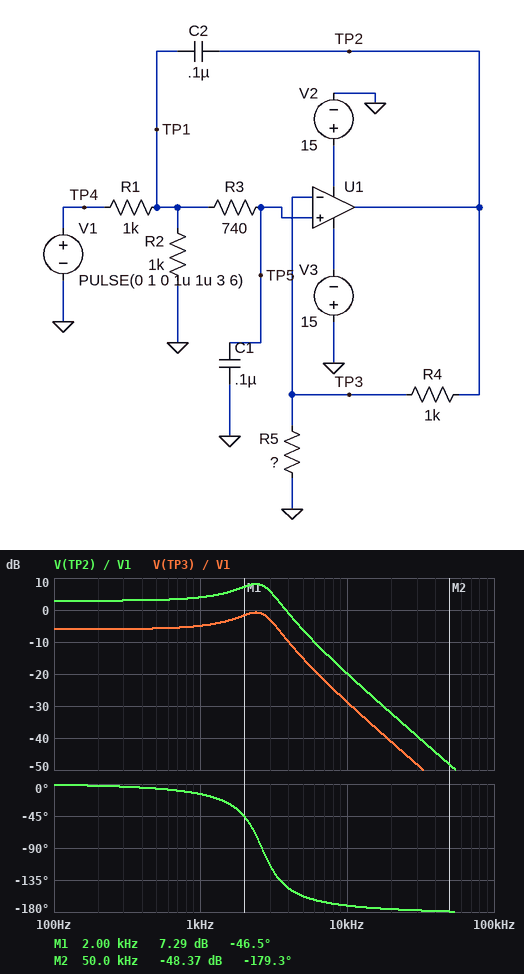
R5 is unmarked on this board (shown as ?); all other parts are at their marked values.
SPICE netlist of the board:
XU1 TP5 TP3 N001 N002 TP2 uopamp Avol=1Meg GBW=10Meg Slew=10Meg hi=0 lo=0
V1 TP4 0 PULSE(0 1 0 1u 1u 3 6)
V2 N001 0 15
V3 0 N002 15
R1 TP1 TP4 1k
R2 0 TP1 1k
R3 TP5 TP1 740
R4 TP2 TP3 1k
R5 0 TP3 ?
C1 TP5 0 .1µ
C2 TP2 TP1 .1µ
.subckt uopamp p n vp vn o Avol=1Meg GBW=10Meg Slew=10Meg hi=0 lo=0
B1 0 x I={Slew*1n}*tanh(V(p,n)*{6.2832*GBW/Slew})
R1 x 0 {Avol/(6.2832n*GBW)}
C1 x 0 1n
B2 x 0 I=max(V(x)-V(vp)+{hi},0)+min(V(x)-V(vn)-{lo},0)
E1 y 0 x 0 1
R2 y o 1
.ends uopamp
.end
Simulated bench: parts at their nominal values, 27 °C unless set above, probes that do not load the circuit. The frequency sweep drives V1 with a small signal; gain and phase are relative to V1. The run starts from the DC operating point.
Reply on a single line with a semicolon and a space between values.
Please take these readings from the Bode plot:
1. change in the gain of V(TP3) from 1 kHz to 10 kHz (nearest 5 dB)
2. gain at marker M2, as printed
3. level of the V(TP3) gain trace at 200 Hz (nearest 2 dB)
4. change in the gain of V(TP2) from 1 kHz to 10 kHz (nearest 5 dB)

-25 dB; -48.37 dB; -6 dB; -25 dB
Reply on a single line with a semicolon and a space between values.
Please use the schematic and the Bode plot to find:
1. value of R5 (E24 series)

560 Ω
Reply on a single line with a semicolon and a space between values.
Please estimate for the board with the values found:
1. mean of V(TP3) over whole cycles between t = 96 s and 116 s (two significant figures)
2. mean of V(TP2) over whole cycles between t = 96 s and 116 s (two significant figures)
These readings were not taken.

250 mV; 700 mV
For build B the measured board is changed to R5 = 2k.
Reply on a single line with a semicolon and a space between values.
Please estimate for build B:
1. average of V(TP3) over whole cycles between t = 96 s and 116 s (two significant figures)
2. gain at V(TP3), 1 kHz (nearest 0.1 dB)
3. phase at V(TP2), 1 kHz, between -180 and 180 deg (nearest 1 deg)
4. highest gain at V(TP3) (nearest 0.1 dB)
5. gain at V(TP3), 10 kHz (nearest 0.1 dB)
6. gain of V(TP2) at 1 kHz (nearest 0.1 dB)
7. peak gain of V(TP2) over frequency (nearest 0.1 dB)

250 mV; -6.5 dB; -36 deg; -6.0 dB; -29.5 dB; -3.0 dB; -2.5 dB
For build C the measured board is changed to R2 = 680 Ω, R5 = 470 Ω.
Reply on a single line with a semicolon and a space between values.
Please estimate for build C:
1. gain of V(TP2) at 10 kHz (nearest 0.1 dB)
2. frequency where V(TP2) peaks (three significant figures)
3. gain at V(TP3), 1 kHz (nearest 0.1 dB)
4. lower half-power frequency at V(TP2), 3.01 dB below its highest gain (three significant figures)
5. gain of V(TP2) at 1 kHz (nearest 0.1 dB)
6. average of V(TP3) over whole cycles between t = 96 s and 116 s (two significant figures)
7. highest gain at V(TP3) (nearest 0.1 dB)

-18.8 dB; 2.70 kHz; -6.9 dB; 1.76 kHz; 3.0 dB; 200 mV; -1.8 dB
